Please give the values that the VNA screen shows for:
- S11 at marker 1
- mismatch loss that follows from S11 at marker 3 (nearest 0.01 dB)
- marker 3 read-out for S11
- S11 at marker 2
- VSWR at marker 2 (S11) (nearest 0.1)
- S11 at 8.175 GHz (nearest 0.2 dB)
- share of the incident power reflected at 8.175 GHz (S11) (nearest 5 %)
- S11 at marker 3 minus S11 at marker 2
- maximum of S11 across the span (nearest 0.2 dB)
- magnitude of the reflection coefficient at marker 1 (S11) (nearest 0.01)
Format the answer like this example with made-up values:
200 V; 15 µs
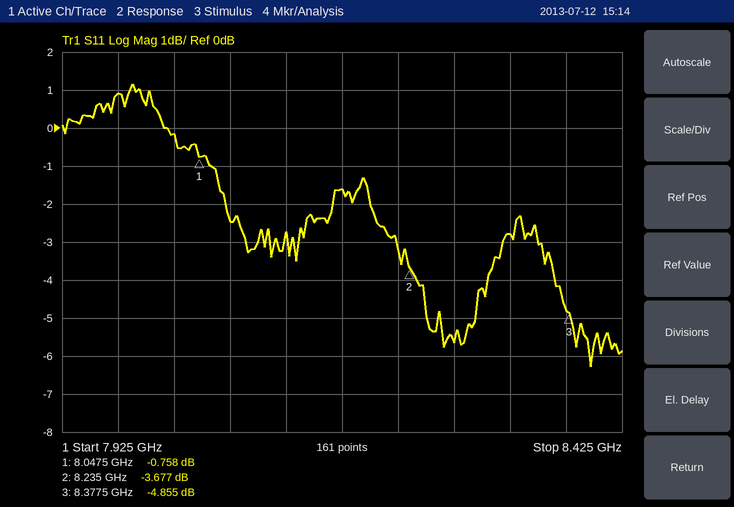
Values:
-0.758 dB; 1.72 dB; -4.855 dB; -3.677 dB; 4.8; -1.6 dB; 70 %; -1.178 dB; 1.2 dB; 0.92
